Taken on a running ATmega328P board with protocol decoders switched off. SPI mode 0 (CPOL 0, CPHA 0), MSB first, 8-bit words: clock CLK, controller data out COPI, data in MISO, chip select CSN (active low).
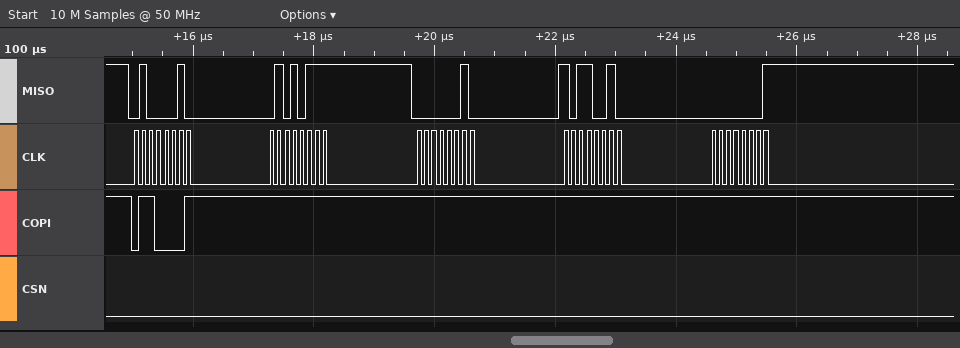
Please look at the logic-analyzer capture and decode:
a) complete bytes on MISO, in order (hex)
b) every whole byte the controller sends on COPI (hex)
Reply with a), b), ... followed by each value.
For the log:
a) 42 57 02 B2 01
b) 61 FF FF FF FF
